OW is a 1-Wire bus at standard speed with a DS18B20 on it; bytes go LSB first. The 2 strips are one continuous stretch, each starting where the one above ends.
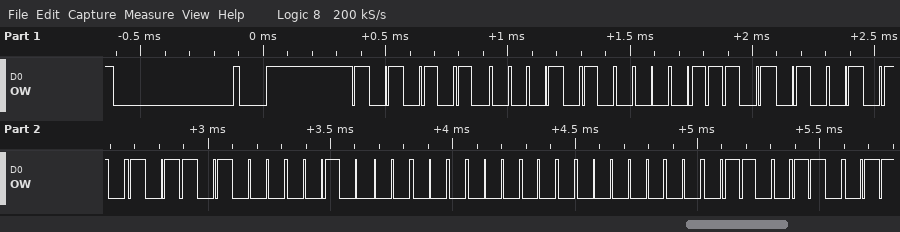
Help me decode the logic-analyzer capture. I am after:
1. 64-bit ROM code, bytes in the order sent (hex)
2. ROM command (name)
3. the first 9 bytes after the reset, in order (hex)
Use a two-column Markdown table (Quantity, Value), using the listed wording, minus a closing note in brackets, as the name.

| Quantity | Value |
|---|---|
| 64-bit ROM code, bytes in the order sent | 28 B8 52 2D 08 00 00 66 |
| ROM command | Match ROM |
| the first 9 bytes after the reset, in order | 55 28 B8 52 2D 08 00 00 66 |
